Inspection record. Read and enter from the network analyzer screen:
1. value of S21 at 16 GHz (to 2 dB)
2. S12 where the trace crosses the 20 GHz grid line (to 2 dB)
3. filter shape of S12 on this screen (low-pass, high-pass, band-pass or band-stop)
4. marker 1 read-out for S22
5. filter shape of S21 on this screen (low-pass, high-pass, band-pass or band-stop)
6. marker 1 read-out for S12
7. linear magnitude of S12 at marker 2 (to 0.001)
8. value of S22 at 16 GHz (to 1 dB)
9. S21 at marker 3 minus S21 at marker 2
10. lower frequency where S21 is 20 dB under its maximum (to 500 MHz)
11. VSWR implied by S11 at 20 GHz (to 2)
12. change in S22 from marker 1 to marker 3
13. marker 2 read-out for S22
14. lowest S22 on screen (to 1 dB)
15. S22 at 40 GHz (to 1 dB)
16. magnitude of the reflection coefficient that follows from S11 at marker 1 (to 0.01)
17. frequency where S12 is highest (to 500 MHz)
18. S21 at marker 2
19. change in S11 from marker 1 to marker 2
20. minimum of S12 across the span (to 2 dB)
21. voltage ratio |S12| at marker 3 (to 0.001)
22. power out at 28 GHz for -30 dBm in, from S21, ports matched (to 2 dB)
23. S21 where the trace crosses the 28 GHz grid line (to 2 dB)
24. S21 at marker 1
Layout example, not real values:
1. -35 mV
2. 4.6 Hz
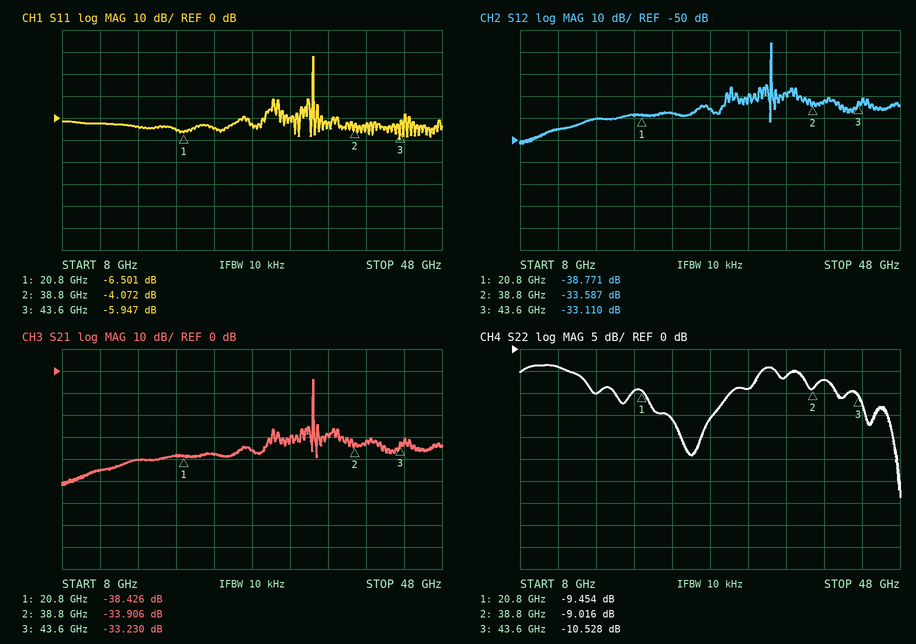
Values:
1. -40 dB
2. -38 dB
3. band-pass
4. -9.454 dB
5. band-pass
6. -38.771 dB
7. 0.021
8. -10 dB
9. 0.676 dB
10. 34.5 GHz
11. 4
12. -1.074 dB
13. -9.016 dB
14. -34 dB
15. -7 dB
16. 0.47
17. 34.5 GHz
18. -33.906 dB
19. 2.429 dB
20. -52 dB
21. 0.022
22. -66 dBm
23. -36 dB
24. -38.426 dB
